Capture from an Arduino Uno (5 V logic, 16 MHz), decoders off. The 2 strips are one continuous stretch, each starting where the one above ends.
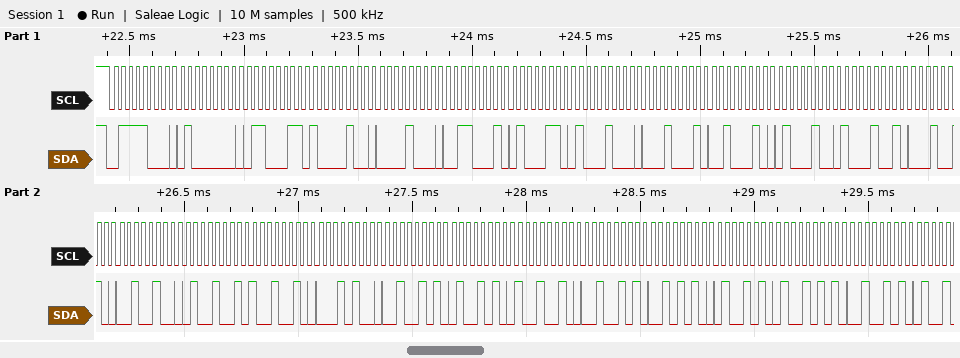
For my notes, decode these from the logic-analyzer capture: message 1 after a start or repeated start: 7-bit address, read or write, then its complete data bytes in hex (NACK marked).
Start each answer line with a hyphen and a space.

- 0x3C write: 40 63 84 08 31 46 88 11 22 44 89 12 24 49 92 14 25 4A 92 25 2A 4A 95 25
